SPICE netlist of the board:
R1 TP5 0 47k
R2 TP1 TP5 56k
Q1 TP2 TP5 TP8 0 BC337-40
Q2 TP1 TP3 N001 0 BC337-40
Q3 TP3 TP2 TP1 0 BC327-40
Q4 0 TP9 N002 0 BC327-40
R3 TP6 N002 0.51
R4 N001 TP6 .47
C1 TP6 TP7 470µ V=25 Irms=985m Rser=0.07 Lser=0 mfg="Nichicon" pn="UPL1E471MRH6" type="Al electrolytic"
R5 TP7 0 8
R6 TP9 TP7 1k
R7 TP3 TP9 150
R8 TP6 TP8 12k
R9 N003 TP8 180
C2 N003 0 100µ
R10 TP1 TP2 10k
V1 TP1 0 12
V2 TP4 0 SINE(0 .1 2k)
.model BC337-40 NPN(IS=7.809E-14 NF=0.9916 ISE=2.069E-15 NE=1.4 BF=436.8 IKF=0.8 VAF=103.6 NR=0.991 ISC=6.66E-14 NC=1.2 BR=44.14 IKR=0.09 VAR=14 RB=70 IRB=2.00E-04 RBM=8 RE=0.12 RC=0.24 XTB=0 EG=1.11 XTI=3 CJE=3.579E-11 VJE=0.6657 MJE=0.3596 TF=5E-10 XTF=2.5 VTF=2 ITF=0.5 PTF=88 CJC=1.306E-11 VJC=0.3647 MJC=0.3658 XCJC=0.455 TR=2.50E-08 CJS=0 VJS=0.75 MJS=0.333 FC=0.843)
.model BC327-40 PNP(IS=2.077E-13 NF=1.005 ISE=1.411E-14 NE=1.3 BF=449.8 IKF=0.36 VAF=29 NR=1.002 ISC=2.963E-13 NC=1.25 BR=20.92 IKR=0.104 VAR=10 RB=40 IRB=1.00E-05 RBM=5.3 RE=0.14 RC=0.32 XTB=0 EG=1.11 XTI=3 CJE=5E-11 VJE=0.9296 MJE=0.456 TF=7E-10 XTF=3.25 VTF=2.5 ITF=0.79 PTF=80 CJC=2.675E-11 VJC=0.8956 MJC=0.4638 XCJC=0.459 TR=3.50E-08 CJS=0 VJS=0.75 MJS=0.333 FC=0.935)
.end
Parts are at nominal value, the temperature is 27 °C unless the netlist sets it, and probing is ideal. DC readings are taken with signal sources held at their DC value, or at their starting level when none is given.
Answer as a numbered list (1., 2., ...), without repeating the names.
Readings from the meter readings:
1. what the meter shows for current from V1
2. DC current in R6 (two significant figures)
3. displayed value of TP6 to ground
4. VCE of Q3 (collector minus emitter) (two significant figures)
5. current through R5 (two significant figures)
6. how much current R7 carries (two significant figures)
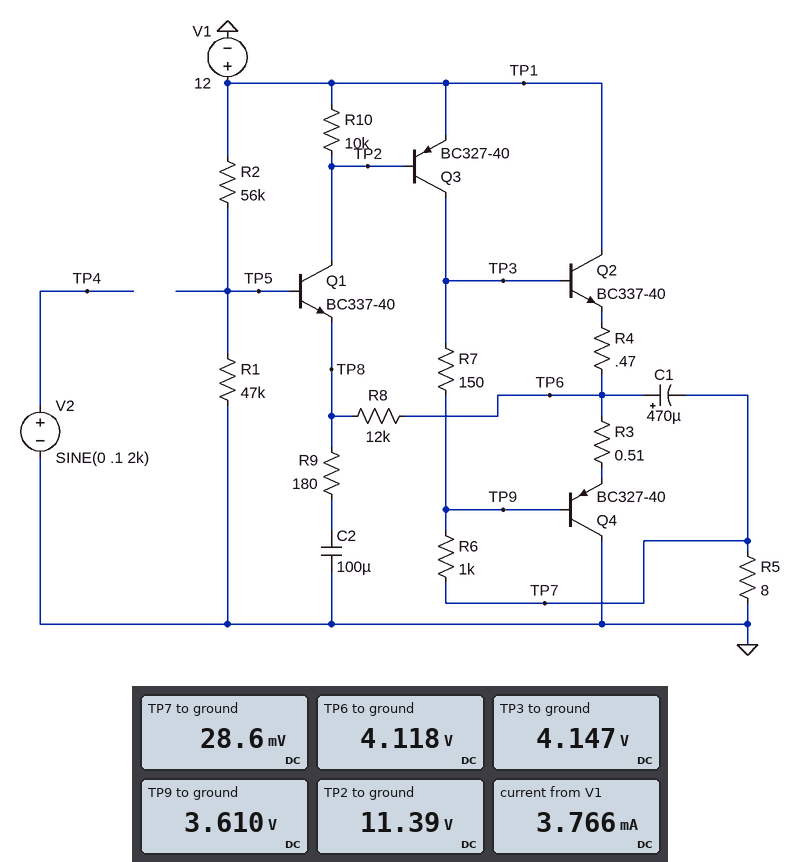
1. 3.766 mA
2. 3.6 mA
3. 4.118 V
4. -7.9 V
5. 3.6 mA
6. 3.6 mA
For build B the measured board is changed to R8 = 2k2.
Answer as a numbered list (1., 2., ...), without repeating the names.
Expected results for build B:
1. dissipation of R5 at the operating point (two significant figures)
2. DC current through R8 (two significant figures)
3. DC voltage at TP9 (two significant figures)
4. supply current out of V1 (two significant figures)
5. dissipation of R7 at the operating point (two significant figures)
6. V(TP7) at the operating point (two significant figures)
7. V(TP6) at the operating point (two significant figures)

1. 140 µW
2. 71 µA
3. 4.3 V
4. 4.4 mA
5. 2.7 mW
6. 34 mV
7. 4.8 V
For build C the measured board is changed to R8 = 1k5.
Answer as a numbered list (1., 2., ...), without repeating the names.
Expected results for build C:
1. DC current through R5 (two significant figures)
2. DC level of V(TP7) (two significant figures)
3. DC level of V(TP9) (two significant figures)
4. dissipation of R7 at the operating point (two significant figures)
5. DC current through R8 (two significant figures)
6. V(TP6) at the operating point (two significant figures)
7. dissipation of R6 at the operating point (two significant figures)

1. 4.3 mA
2. 34 mV
3. 4.3 V
4. 2.8 mW
5. 71 µA
6. 4.8 V
7. 18 mW
